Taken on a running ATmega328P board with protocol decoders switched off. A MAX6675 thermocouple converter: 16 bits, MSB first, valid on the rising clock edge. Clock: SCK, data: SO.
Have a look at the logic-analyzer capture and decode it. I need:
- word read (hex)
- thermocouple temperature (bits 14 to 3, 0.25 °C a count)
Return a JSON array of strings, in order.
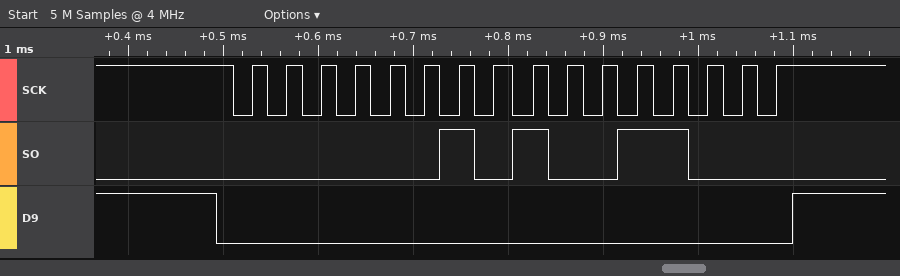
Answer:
["0x0298", "20.75 °C"]
